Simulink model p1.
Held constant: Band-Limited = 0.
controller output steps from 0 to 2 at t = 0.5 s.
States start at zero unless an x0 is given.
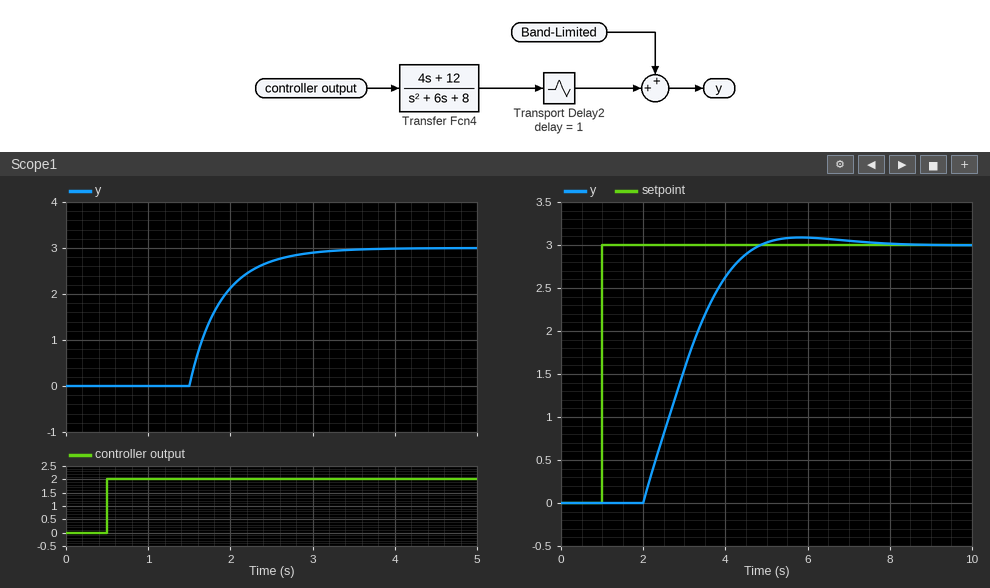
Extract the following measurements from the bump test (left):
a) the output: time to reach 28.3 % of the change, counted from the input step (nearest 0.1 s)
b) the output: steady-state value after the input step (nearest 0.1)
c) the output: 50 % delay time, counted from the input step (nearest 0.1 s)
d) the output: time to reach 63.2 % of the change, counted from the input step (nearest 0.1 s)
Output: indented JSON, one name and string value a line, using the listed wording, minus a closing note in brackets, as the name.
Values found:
{
  "the output: time to reach 28.3 % of the change, counted from the input step": "1.1 s",
  "the output: steady-state value after the input step": "3.0",
  "the output: 50 % delay time, counted from the input step": "1.3 s",
  "the output: time to reach 63.2 % of the change, counted from the input step": "1.4 s"
}
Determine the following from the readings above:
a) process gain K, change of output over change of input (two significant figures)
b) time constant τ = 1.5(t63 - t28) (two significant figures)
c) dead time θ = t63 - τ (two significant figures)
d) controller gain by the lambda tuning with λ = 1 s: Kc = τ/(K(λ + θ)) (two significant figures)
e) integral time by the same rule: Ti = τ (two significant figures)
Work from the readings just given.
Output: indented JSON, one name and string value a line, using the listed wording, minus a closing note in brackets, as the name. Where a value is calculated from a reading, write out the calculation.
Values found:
{
  "process gain K, change of output over change of input": "(3 - 0) / 2 = 1.5",
  "time constant τ = 1.5(t63 - t28)": "1.5 × (1.4 - 1.1) = 0.45 s",
  "dead time θ = t63 - τ": "1.4 - 0.45 = 0.95 s",
  "controller gain by the lambda tuning with λ = 1 s: Kc = τ/(K(λ + θ))": "0.45 / (1.5 × (1 + 0.95)) = 0.15",
  "integral time by the same rule: Ti = τ": "0.45 s"
}
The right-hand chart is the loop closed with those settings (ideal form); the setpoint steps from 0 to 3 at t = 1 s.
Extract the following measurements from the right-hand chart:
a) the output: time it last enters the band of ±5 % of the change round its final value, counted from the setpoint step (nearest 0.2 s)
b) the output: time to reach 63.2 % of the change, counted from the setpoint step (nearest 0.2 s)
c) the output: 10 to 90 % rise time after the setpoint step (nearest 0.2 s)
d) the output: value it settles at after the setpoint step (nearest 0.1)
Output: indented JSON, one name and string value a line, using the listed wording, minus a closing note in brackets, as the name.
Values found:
{
  "the output: time it last enters the band of ±5 % of the change round its final value, counted from the setpoint step": "3.4 s",
  "the output: time to reach 63.2 % of the change, counted from the setpoint step": "2.2 s",
  "the output: 10 to 90 % rise time after the setpoint step": "2.0 s",
  "the output: value it settles at after the setpoint step": "3.0"
}
